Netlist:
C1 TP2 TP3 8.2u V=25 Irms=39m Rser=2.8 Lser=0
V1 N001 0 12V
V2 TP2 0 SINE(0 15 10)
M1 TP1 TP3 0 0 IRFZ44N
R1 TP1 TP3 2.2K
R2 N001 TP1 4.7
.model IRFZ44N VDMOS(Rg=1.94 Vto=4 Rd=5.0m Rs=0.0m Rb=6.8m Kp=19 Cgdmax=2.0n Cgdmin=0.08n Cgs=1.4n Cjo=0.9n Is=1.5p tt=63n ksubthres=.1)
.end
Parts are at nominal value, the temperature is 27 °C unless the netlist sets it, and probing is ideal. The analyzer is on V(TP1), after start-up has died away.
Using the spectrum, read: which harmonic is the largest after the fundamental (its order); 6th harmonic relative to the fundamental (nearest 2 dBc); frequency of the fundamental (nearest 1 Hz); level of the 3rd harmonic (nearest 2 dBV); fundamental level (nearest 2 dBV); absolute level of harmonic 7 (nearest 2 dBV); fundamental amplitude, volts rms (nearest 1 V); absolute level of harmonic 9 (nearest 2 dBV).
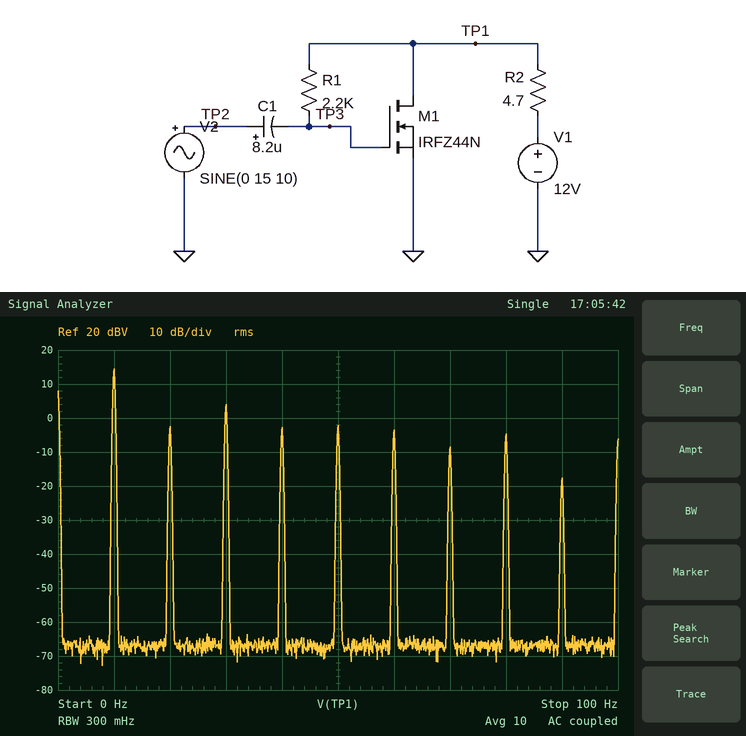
3
-18 dBc
10 Hz
4 dBV
14 dBV
-8 dBV
5 V
-18 dBV
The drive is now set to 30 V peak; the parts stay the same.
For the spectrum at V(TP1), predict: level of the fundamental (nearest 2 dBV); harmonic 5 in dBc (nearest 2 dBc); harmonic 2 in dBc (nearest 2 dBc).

14 dBV
-14 dBc
-24 dBc
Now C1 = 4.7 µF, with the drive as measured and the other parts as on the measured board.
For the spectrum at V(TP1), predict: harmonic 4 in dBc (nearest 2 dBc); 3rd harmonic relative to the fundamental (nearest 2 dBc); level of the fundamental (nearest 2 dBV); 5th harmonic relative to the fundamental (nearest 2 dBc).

-22 dBc
-16 dBc
14 dBV
-30 dBc
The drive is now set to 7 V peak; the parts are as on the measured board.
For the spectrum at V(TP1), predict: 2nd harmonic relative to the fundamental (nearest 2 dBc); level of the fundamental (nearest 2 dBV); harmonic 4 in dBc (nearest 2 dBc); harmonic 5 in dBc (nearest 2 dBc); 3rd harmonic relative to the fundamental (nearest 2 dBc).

-14 dBc
14 dBV
-26 dBc
-26 dBc
-18 dBc
